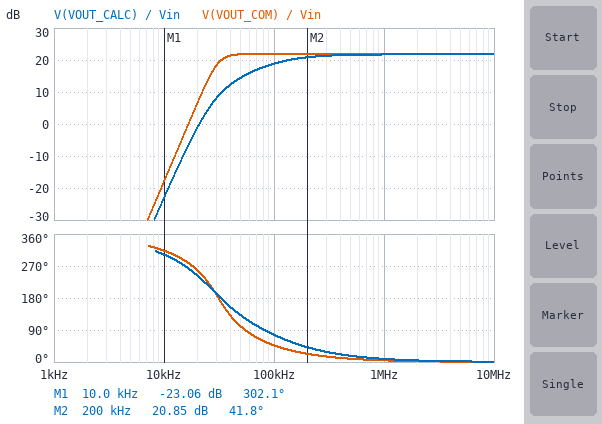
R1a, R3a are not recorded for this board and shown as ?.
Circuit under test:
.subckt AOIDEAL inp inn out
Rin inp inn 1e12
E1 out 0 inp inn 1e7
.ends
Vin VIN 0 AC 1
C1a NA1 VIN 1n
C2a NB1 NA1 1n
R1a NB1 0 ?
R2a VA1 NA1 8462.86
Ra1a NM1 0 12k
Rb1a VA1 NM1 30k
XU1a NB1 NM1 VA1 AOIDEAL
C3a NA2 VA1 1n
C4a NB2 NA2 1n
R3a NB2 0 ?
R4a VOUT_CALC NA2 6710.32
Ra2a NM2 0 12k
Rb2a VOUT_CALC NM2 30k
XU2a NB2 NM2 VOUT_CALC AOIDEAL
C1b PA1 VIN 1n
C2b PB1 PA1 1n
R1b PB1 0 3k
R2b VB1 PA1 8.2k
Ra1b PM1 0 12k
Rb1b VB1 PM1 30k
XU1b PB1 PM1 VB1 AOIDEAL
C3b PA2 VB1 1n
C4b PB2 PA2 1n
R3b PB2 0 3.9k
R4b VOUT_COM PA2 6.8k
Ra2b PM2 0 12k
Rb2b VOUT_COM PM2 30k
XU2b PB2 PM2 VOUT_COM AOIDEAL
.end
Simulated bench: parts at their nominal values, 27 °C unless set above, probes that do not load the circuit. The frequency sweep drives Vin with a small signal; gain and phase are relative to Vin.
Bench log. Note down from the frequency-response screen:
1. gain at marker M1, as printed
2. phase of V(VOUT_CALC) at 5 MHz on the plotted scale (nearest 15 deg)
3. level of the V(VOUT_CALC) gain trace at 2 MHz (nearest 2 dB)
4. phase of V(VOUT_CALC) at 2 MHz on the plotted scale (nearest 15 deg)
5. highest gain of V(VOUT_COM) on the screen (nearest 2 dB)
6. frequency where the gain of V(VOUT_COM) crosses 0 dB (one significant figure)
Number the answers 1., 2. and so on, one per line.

1. -23.06 dB
2. 0 deg
3. 22 dB
4. 0 deg
5. 22 dB
6. 20 kHz
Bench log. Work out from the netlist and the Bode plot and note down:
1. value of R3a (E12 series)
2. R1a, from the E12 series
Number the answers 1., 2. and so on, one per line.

1. 1.8 kΩ
2. 3.9 kΩ
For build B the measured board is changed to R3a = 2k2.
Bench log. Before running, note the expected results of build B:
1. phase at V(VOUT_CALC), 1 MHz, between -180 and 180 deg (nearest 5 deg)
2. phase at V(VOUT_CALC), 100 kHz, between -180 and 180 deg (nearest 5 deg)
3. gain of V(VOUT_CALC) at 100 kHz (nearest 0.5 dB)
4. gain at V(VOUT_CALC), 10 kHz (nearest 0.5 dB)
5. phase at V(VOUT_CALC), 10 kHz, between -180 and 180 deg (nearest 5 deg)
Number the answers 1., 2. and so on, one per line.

1. 5 deg
2. 65 deg
3. 20.5 dB
4. -21.0 dB
5. -55 deg
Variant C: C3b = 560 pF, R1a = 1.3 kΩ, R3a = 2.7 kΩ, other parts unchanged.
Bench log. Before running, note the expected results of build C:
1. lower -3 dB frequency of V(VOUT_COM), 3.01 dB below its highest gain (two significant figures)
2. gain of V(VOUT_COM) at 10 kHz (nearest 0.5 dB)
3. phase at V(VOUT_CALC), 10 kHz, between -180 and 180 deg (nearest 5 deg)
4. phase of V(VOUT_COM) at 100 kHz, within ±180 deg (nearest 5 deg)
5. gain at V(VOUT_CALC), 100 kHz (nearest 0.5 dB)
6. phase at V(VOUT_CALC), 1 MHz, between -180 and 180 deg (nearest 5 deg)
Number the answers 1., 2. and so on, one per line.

1. 38 kHz
2. -23.0 dB
3. -65 deg
4. 40 deg
5. 15.0 dB
6. 15 deg
